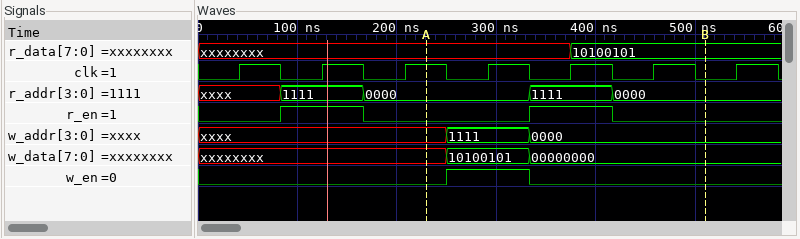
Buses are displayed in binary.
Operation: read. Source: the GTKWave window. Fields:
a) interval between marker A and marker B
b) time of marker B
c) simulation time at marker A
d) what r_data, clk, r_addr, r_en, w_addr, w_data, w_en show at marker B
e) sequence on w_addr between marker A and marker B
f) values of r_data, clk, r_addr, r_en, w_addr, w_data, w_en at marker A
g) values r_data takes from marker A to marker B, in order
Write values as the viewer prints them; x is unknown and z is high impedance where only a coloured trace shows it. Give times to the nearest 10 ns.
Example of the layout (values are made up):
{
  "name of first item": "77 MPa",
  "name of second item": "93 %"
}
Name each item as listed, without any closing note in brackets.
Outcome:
{
  "interval between marker A and marker B": "280 ns",
  "time of marker B": "510 ns",
  "simulation time at marker A": "230 ns",
  "what r_data, clk, r_addr, r_en, w_addr, w_data, w_en show at marker B": "r_data=10100101, clk=0, r_addr=0000, r_en=0, w_addr=0000, w_data=00000000, w_en=0",
  "sequence on w_addr between marker A and marker B": "xxxx, 1111, 0000",
  "values of r_data, clk, r_addr, r_en, w_addr, w_data, w_en at marker A": "r_data=xxxxxxxx, clk=1, r_addr=0000, r_en=0, w_addr=xxxx, w_data=xxxxxxxx, w_en=0",
  "values r_data takes from marker A to marker B, in order": "xxxxxxxx, 10100101"
}
